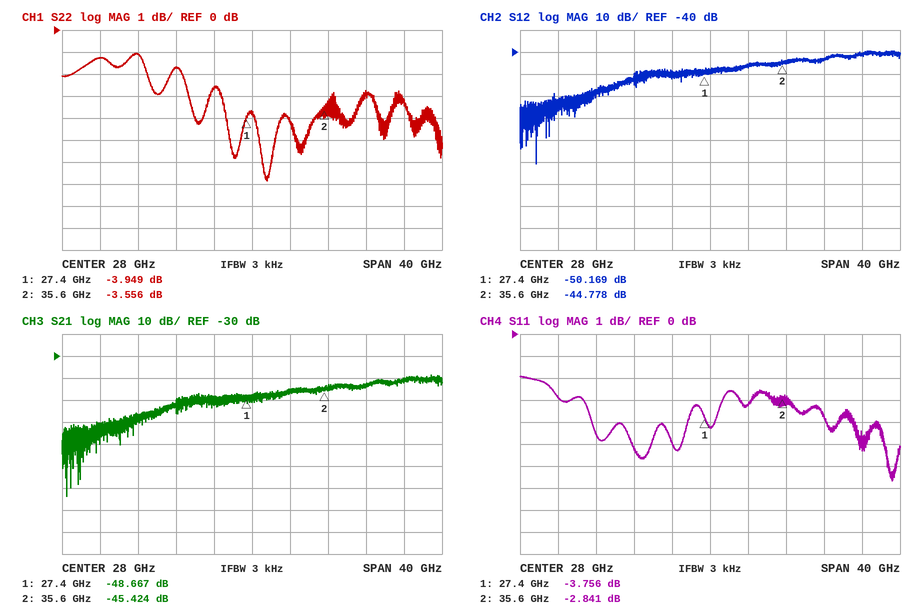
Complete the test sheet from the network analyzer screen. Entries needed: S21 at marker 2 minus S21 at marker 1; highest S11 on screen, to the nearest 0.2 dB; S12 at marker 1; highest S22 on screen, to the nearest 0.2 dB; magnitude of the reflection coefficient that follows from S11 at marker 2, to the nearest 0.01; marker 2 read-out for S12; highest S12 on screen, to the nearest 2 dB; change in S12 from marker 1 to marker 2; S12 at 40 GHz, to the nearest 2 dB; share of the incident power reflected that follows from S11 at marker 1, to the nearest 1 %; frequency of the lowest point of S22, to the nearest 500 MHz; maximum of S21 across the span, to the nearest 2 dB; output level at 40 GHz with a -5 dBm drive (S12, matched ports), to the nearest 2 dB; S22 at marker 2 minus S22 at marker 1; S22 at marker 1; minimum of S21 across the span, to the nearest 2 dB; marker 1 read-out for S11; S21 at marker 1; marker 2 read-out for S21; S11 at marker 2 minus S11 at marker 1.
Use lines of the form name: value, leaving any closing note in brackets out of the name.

S21 at marker 2 minus S21 at marker 1: 3.243 dB
highest S11 on screen, to the nearest 0.2 dB: -2.0 dB
S12 at marker 1: -50.169 dB
highest S22 on screen, to the nearest 0.2 dB: -1.0 dB
magnitude of the reflection coefficient that follows from S11 at marker 2, to the nearest 0.01: 0.72
marker 2 read-out for S12: -44.778 dB
highest S12 on screen, to the nearest 2 dB: -40 dB
change in S12 from marker 1 to marker 2: 5.391 dB
S12 at 40 GHz, to the nearest 2 dB: -44 dB
share of the incident power reflected that follows from S11 at marker 1, to the nearest 1 %: 42 %
frequency of the lowest point of S22, to the nearest 500 MHz: 29.5 GHz
maximum of S21 across the span, to the nearest 2 dB: -38 dB
output level at 40 GHz with a -5 dBm drive (S12, matched ports), to the nearest 2 dB: -48 dBm
S22 at marker 2 minus S22 at marker 1: 0.393 dB
S22 at marker 1: -3.949 dB
minimum of S21 across the span, to the nearest 2 dB: -94 dB
marker 1 read-out for S11: -3.756 dB
S21 at marker 1: -48.667 dB
marker 2 read-out for S21: -45.424 dB
S11 at marker 2 minus S11 at marker 1: 0.915 dB
